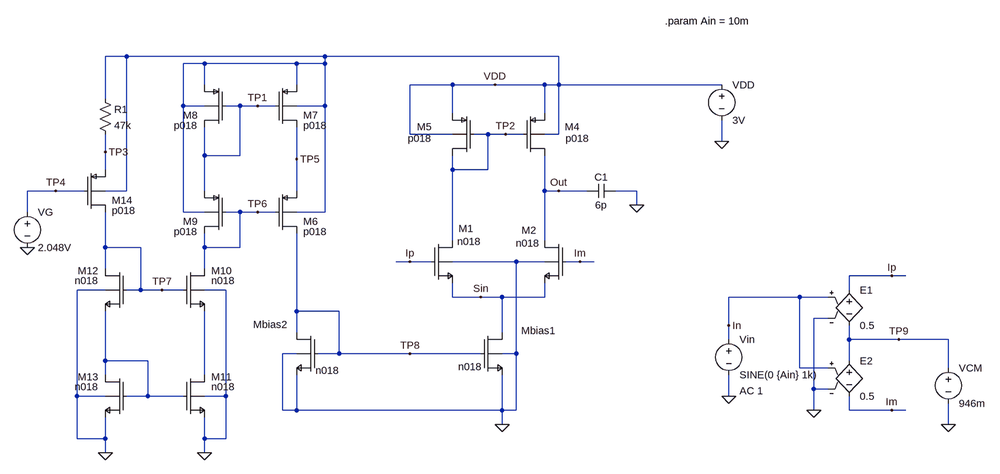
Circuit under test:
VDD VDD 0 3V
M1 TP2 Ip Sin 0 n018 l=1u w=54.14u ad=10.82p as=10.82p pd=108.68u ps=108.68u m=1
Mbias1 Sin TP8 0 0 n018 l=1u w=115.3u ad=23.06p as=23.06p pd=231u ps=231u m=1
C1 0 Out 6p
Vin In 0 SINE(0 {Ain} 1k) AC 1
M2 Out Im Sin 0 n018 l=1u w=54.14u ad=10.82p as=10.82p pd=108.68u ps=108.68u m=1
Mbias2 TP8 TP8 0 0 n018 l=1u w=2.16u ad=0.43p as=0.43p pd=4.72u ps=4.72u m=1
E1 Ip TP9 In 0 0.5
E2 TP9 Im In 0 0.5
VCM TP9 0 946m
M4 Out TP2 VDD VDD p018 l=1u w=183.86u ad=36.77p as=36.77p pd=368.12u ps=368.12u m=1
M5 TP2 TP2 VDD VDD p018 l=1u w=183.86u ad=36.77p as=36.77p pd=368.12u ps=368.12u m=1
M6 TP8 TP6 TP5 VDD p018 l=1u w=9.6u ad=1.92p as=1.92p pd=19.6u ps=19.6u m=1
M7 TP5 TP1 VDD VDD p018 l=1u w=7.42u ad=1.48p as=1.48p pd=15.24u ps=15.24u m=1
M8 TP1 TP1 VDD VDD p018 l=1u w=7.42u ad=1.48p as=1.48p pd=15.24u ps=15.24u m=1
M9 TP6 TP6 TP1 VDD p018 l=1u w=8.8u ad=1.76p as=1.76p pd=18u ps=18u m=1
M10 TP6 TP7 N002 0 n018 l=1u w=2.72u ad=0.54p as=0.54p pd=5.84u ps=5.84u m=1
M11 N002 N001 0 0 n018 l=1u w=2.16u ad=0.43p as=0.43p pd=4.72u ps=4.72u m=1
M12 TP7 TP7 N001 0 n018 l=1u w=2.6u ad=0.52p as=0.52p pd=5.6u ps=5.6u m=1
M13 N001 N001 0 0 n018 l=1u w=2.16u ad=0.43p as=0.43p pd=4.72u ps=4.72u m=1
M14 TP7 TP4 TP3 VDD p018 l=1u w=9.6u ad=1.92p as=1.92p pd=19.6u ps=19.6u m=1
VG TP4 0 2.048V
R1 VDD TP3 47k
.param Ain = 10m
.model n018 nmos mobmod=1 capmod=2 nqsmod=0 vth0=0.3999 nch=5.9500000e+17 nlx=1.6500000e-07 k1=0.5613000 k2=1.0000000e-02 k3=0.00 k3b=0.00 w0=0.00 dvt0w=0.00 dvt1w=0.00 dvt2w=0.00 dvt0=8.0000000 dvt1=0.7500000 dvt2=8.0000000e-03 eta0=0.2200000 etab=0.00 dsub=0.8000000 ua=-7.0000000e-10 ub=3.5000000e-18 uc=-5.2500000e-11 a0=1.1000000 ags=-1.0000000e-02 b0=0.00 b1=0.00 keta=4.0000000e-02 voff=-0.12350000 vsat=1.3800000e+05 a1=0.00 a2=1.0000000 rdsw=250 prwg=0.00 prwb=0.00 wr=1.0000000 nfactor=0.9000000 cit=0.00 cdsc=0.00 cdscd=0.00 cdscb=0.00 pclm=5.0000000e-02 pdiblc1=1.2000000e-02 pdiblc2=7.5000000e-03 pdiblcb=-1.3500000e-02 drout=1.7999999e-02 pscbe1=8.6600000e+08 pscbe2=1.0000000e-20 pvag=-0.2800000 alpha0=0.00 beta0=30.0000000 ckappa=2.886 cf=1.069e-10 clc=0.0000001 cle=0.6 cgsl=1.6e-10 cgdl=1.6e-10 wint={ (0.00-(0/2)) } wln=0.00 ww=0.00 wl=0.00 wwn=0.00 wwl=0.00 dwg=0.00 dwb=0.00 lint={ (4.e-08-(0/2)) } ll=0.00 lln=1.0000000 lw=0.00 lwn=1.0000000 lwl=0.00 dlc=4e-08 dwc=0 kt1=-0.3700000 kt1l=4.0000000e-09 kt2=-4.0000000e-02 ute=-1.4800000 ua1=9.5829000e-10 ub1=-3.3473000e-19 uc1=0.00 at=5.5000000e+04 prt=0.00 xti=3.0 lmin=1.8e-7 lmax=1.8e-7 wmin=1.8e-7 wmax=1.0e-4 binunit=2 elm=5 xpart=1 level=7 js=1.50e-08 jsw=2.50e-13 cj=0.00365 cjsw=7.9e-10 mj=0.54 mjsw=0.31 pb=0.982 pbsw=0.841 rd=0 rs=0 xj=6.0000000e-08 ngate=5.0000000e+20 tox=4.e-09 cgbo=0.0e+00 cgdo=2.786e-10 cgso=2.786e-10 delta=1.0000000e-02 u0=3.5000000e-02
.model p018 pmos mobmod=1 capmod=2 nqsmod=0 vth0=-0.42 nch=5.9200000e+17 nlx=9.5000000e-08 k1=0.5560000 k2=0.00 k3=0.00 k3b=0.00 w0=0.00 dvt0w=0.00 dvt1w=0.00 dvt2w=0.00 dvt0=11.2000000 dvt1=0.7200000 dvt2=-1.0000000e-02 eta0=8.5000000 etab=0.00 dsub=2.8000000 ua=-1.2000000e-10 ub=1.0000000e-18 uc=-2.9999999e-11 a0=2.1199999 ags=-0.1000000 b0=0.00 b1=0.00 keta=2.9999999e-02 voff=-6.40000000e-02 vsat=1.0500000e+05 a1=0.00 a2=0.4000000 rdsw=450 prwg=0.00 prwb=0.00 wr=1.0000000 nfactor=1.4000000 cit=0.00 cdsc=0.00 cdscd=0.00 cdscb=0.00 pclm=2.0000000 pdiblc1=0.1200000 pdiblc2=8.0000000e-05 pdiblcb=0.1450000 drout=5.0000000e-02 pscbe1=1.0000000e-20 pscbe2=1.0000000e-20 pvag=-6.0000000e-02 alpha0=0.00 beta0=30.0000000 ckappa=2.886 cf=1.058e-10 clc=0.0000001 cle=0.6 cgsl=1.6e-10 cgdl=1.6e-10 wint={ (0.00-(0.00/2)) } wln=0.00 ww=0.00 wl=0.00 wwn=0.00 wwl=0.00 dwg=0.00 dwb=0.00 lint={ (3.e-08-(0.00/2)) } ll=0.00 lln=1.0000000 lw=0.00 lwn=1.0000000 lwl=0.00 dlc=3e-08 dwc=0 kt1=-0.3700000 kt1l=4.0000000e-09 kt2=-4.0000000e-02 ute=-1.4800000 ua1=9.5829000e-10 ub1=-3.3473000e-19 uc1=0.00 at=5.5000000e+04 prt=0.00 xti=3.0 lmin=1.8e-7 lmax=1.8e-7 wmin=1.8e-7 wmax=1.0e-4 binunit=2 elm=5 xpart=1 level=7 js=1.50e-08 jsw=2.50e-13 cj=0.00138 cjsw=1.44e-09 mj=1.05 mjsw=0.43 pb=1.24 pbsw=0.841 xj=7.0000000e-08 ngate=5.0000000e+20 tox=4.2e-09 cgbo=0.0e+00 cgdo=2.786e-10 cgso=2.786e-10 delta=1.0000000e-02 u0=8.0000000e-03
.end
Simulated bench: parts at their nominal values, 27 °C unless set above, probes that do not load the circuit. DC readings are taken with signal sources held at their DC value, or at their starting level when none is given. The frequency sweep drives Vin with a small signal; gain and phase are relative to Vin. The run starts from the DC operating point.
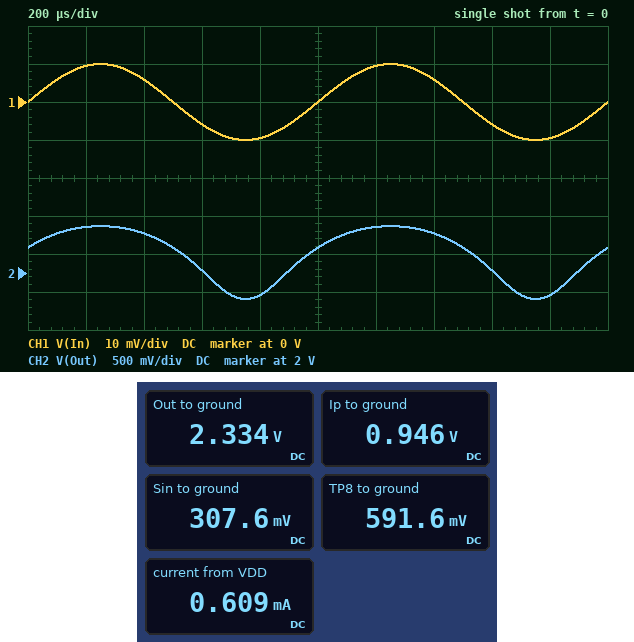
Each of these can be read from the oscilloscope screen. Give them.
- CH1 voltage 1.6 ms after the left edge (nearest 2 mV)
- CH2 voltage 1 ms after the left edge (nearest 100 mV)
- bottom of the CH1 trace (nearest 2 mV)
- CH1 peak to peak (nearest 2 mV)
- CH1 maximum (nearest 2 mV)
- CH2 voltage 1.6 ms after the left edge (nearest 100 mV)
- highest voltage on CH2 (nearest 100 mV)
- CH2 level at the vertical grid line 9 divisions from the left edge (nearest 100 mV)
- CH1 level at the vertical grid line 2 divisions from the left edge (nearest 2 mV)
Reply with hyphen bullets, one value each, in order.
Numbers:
- -6 mV
- 2.3 V
- -10 mV
- 20 mV
- 10 mV
- 2.0 V
- 2.6 V
- 1.7 V
- 6 mV
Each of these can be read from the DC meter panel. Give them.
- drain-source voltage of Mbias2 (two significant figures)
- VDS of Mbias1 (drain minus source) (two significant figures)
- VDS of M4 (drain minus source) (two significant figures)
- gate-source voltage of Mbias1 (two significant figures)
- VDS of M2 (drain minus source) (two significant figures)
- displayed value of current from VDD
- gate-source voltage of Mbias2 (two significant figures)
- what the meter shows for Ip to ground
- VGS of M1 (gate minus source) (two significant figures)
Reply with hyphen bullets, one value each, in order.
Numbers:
- 590 mV
- 310 mV
- -670 mV
- 590 mV
- 2.0 V
- 0.609 mA
- 590 mV
- 0.946 V
- 640 mV
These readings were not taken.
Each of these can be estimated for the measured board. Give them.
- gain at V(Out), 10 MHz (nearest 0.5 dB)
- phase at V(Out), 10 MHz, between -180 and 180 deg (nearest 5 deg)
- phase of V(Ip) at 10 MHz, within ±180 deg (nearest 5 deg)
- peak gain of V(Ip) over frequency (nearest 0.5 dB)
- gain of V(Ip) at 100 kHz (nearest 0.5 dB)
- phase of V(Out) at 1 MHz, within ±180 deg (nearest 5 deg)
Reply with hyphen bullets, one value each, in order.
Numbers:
- 14.0 dB
- -85 deg
- 0 deg
- -6.0 dB
- -6.0 dB
- -35 deg
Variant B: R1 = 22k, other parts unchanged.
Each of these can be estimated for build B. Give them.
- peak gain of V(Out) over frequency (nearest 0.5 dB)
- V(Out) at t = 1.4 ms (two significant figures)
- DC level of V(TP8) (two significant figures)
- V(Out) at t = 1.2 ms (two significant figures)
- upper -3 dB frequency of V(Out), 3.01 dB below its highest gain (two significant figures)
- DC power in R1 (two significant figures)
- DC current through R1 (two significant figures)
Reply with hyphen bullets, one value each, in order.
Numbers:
- 31.0 dB
- 2.4 V
- 660 mV
- 2.5 V
- 1.7 MHz
- 3.0 µW
- 12 µA
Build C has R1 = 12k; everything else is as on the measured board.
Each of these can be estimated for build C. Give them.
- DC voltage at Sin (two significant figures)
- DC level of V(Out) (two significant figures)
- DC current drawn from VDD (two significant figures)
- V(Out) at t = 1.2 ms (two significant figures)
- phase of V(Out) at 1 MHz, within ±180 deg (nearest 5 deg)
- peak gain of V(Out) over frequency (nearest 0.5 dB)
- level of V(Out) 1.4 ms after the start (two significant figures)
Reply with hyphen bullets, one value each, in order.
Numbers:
- 220 mV
- 2.2 V
- 1.1 mA
- 2.5 V
- -30 deg
- 30.5 dB
- 2.4 V
